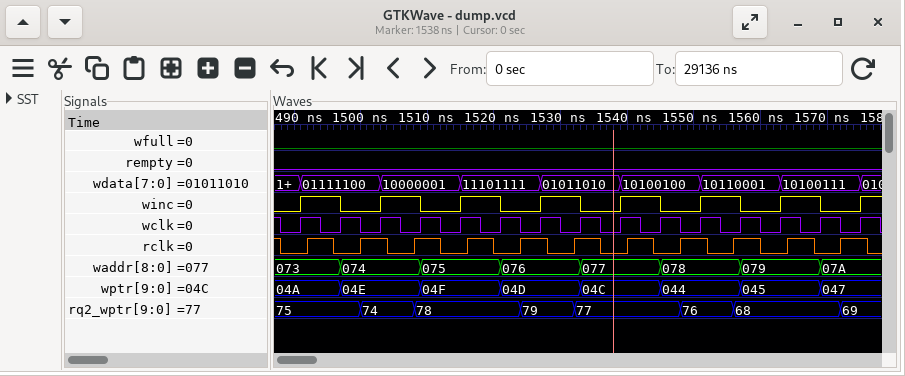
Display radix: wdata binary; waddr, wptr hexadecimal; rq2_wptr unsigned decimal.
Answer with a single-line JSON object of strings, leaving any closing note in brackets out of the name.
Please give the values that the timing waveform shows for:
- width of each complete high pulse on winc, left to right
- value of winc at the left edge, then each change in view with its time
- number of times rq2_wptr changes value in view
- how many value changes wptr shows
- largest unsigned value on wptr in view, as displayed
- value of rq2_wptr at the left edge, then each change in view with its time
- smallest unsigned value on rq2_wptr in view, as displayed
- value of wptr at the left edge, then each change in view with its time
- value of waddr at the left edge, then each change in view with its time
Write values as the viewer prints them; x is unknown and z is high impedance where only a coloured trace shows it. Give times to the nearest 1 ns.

{"width of each complete high pulse on winc, left to right": "6 ns, 6 ns, 6 ns, 6 ns, 6 ns, 6 ns, 6 ns", "value of winc at the left edge, then each change in view with its time": "0, 1 at 1491 ns, 0 at 1497 ns, 1 at 1503 ns, 0 at 1509 ns, 1 at 1515 ns, 0 at 1521 ns, 1 at 1527 ns, 0 at 1533 ns, 1 at 1539 ns, 0 at 1545 ns, 1 at 1551 ns, 0 at 1557 ns, 1 at 1563 ns, 0 at 1569 ns, 1 at 1575 ns", "number of times rq2_wptr changes value in view": "7", "how many value changes wptr shows": "7", "largest unsigned value on wptr in view, as displayed": "04F", "value of rq2_wptr at the left edge, then each change in view with its time": "75, 74 at 1500 ns, 78 at 1508 ns, 79 at 1524 ns, 77 at 1532 ns, 76 at 1548 ns, 68 at 1556 ns, 69 at 1572 ns", "smallest unsigned value on rq2_wptr in view, as displayed": "68", "value of wptr at the left edge, then each change in view with its time": "04A, 04E at 1497 ns, 04F at 1509 ns, 04D at 1521 ns, 04C at 1533 ns, 044 at 1545 ns, 045 at 1557 ns, 047 at 1569 ns", "value of waddr at the left edge, then each change in view with its time": "073, 074 at 1497 ns, 075 at 1509 ns, 076 at 1521 ns, 077 at 1533 ns, 078 at 1545 ns, 079 at 1557 ns, 07A at 1569 ns"}
